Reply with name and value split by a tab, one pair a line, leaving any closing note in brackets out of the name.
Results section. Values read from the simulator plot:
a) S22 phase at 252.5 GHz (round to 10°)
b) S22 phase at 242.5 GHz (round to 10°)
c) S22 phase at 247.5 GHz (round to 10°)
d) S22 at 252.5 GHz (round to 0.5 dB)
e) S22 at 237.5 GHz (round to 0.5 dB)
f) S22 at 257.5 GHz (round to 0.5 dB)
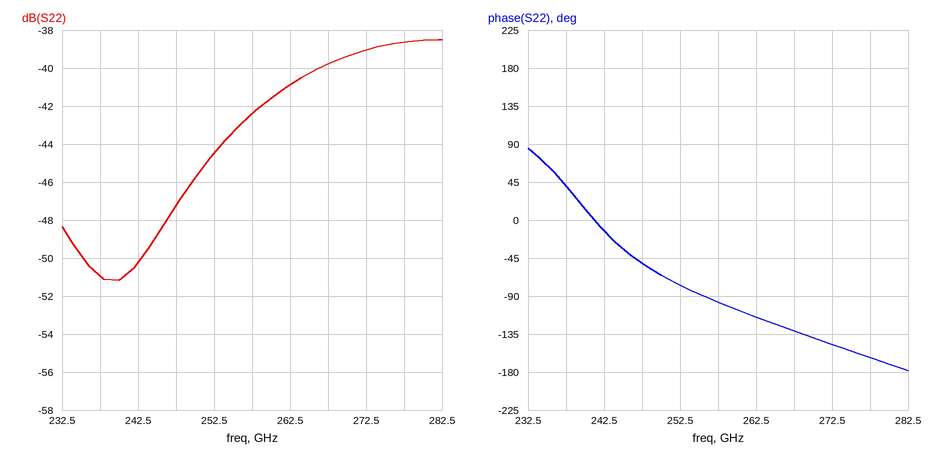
S22 phase at 252.5 GHz	-80°
S22 phase at 242.5 GHz	-10°
S22 phase at 247.5 GHz	-50°
S22 at 252.5 GHz	-44.5 dB
S22 at 237.5 GHz	-51.0 dB
S22 at 257.5 GHz	-42.5 dB
